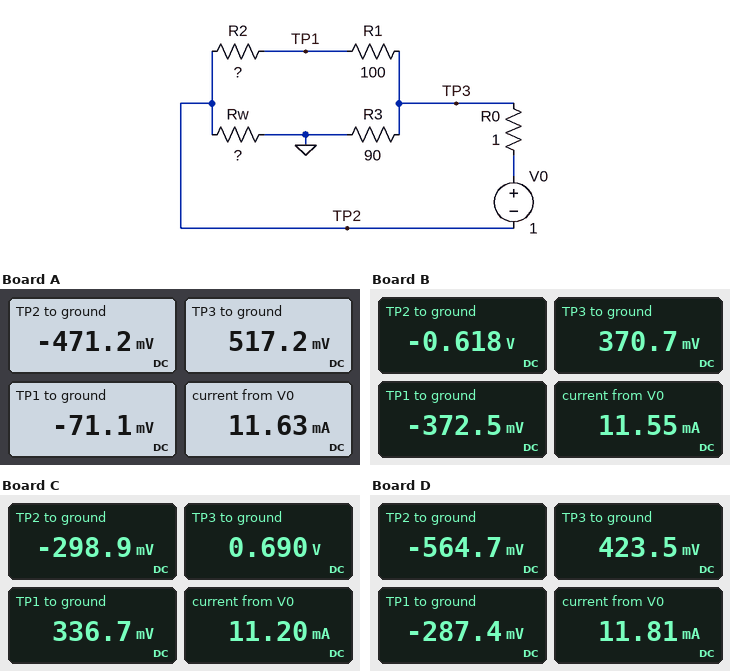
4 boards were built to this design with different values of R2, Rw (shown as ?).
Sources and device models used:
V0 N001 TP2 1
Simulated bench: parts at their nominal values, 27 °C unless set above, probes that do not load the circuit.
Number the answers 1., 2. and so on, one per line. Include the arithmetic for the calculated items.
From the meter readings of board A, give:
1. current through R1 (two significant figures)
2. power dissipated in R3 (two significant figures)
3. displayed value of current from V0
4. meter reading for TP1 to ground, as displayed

1. (517.2 mV - (-71.1 mV)) / 100 Ω = 5.9 mA
2. (517.2 mV)^2 / 90 Ω = 3.0 mW
3. 11.63 mA
4. -71.1 mV
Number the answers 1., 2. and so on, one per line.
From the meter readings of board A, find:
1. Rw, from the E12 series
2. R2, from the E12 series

1. 82 Ω
2. 68 Ω
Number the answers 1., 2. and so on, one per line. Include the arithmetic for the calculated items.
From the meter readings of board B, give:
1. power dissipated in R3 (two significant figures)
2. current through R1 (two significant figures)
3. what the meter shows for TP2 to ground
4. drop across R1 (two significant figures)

1. (370.7 mV)^2 / 90 Ω = 1.5 mW
2. (370.7 mV - (-372.5 mV)) / 100 Ω = 7.4 mA
3. -0.618 V
4. 370.7 mV - (-372.5 mV) = 740 mV
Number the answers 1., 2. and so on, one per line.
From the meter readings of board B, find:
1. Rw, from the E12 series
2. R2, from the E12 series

1. 150 Ω
2. 33 Ω
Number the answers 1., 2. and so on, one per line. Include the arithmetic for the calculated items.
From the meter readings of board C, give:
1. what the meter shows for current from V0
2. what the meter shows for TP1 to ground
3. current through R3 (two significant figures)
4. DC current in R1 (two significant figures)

1. 11.20 mA
2. 336.7 mV
3. (690 mV) / 90 Ω = 7.7 mA
4. (690 mV - 336.7 mV) / 100 Ω = 3.5 mA
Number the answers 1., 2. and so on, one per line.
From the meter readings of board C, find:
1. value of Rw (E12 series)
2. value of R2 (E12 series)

1. 39 Ω
2. 180 Ω
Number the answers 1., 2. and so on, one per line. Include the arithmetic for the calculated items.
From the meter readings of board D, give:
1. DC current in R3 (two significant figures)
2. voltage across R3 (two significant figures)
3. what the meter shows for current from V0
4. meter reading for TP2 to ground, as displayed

1. (423.5 mV) / 90 Ω = 4.7 mA
2. 423.5 mV = 420 mV
3. 11.81 mA
4. -564.7 mV
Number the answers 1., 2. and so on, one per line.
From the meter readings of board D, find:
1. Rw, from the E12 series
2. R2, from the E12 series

1. 120 Ω
2. 39 Ω
